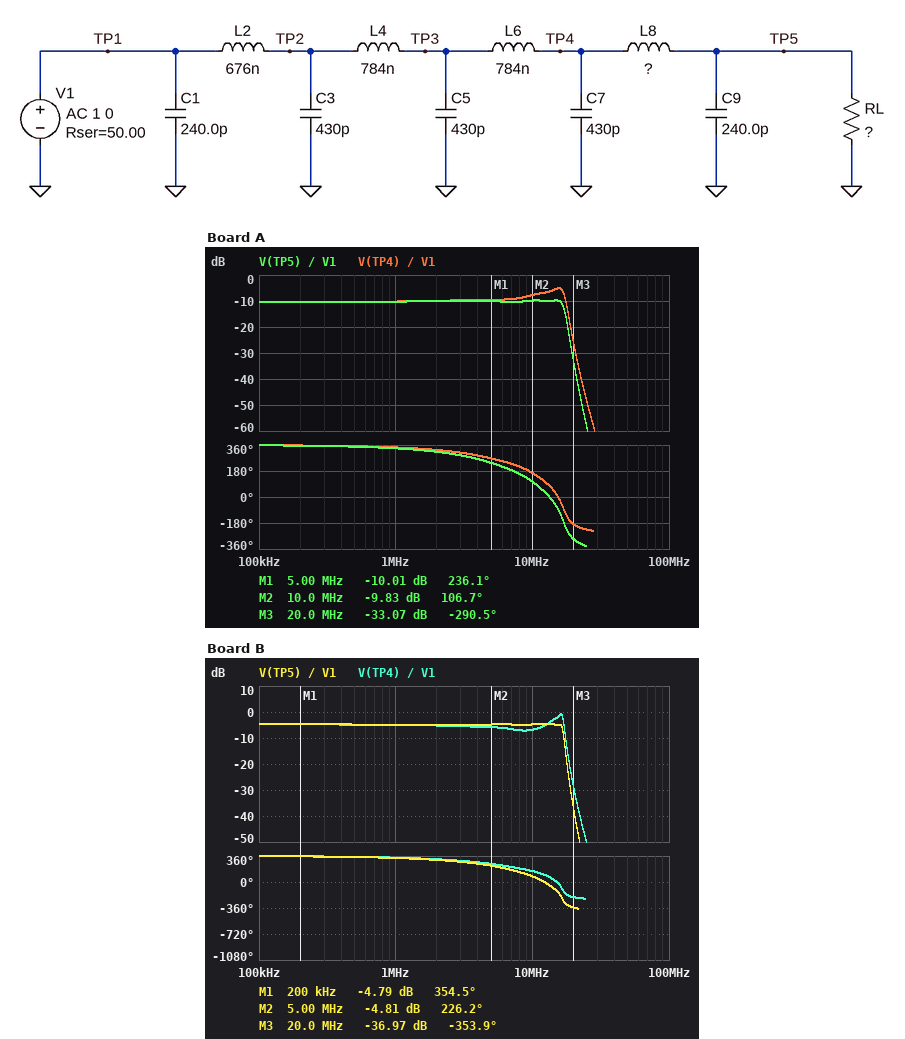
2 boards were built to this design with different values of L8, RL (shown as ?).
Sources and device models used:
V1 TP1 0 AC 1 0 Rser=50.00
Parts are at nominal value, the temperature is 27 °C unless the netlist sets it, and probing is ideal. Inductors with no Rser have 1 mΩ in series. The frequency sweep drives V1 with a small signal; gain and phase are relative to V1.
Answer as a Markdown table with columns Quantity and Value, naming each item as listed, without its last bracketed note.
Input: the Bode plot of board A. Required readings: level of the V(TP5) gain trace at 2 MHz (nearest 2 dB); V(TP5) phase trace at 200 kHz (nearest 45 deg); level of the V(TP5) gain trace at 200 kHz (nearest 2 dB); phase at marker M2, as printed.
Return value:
| Quantity | Value |
|---|---|
| level of the V(TP5) gain trace at 2 MHz | -10 dB |
| V(TP5) phase trace at 200 kHz | 360 deg |
| level of the V(TP5) gain trace at 200 kHz | -10 dB |
| phase at marker M2, as printed | 106.7 deg |
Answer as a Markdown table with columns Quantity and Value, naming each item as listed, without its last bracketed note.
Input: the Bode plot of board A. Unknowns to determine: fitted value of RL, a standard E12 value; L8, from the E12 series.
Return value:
| Quantity | Value |
|---|---|
| fitted value of RL, a standard E12 value | 22 Ω |
| L8, from the E12 series | 390 nH |
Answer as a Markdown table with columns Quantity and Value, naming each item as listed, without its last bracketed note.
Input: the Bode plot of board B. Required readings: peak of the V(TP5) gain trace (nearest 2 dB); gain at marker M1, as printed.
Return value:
| Quantity | Value |
|---|---|
| peak of the V(TP5) gain trace | -4 dB |
| gain at marker M1, as printed | -4.79 dB |
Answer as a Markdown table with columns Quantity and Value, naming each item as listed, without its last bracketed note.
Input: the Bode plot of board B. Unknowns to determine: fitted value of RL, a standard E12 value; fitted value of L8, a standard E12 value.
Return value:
| Quantity | Value |
|---|---|
| fitted value of RL, a standard E12 value | 68 Ω |
| fitted value of L8, a standard E12 value | 820 nH |
